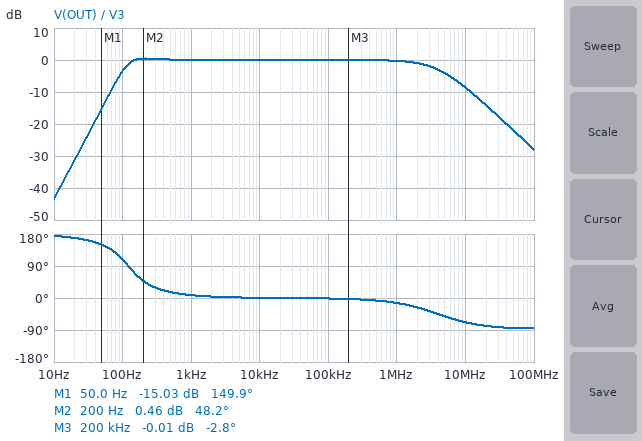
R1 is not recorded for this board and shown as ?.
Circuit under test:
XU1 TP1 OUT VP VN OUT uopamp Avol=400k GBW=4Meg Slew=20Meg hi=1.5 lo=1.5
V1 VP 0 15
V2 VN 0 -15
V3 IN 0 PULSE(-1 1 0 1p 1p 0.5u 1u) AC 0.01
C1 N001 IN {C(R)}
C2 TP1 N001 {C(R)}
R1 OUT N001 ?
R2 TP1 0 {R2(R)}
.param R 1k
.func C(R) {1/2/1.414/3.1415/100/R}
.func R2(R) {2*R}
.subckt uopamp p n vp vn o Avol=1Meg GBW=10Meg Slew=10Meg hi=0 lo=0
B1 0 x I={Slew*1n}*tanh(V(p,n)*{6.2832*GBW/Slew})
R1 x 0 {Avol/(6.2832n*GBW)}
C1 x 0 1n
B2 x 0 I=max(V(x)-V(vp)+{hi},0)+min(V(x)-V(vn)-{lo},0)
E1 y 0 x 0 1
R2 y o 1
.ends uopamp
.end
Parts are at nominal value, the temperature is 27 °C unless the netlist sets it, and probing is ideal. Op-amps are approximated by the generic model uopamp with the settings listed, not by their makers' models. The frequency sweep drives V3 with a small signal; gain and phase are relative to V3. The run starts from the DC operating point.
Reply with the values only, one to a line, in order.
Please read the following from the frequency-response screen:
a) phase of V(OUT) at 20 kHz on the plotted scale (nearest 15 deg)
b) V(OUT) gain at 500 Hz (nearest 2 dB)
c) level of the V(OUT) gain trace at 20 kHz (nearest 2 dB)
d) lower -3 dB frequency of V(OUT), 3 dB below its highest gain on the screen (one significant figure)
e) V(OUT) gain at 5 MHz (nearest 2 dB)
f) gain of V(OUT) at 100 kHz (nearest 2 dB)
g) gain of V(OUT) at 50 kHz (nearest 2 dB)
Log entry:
0 deg
0 dB
0 dB
100 Hz
-4 dB
0 dB
0 dB
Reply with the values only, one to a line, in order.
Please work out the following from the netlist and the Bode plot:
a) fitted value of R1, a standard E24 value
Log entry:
680 Ω
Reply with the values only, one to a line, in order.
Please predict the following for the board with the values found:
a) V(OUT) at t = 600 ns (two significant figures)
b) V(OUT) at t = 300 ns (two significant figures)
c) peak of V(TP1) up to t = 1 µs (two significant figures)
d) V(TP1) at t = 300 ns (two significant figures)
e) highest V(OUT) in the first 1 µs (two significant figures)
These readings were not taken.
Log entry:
380 mV
2.0 V
2.0 V
2.0 V
2.0 V
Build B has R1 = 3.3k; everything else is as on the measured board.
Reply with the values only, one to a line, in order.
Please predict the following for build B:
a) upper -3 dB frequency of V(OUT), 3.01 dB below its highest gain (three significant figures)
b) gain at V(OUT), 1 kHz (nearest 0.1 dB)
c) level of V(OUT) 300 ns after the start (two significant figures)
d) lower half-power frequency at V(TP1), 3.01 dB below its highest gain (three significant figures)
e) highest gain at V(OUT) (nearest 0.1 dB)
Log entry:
4.00 MHz
-0.1 dB
2.0 V
121 Hz
0 dB
